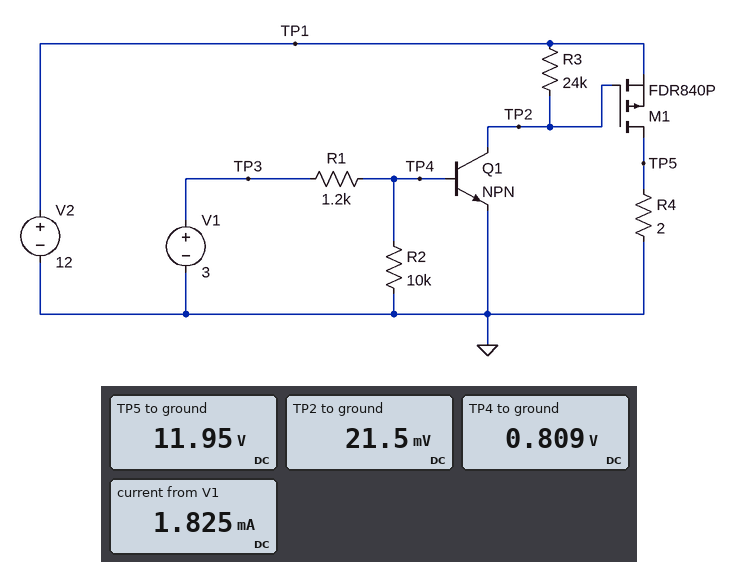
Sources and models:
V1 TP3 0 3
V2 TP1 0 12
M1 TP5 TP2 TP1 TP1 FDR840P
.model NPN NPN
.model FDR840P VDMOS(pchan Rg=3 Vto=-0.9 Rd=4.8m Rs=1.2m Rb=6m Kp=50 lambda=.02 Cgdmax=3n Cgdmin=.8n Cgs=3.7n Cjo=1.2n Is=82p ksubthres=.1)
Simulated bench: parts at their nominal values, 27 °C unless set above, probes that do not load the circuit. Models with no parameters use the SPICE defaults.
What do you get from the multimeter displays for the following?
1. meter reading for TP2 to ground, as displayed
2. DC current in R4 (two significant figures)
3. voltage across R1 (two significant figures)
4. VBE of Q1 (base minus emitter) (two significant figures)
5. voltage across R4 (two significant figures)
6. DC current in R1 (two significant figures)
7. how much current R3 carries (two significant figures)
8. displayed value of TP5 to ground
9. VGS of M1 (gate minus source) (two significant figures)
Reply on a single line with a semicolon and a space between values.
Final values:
21.5 mV; 6.0 A; 2.2 V; 810 mV; 12 V; 1.8 mA; 500 µA; 11.95 V; -12 V
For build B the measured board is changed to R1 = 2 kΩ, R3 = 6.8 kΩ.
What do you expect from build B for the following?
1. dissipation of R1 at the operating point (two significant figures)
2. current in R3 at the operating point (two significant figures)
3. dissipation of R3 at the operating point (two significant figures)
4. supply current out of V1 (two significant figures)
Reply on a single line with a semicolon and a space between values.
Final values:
2.4 mW; 1.8 mA; 21 mW; 1.1 mA
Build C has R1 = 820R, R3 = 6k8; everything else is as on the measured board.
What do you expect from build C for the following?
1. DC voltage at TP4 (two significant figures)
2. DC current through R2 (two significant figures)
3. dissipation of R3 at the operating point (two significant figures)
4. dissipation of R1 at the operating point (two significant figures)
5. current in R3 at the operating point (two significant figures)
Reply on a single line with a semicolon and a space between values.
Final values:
820 mV; 82 µA; 21 mW; 5.8 mW; 1.8 mA
